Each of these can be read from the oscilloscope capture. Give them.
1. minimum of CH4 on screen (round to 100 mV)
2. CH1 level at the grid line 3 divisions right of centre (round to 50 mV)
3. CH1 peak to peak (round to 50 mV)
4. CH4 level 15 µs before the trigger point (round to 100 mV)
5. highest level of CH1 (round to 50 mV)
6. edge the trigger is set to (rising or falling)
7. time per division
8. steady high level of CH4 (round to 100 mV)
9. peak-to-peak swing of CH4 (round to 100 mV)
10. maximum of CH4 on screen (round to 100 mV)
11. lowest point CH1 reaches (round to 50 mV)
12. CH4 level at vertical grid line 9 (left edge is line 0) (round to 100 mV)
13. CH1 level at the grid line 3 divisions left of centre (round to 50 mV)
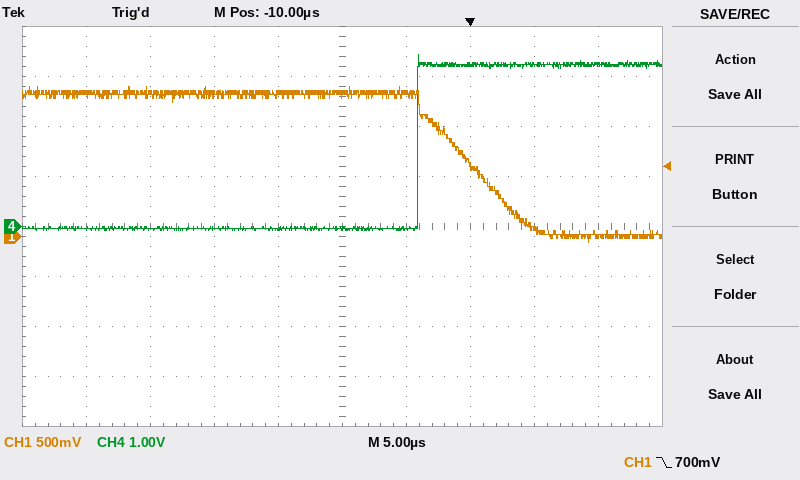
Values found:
-100 mV
50 mV
1.55 V
0.0 V
1.50 V
falling
5 µs
3.2 V
3.5 V
3.4 V
-50 mV
3.2 V
1.40 V
